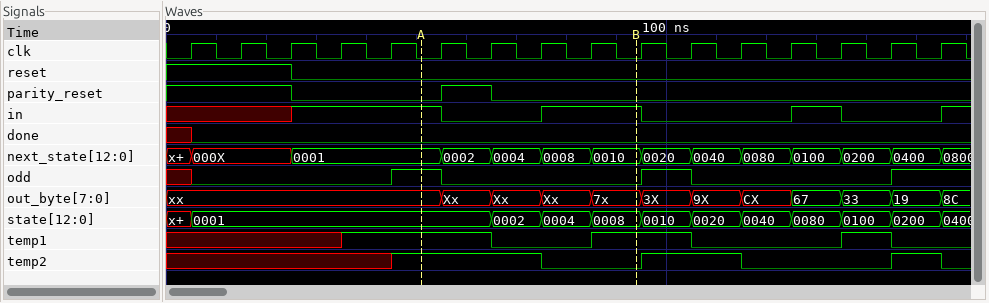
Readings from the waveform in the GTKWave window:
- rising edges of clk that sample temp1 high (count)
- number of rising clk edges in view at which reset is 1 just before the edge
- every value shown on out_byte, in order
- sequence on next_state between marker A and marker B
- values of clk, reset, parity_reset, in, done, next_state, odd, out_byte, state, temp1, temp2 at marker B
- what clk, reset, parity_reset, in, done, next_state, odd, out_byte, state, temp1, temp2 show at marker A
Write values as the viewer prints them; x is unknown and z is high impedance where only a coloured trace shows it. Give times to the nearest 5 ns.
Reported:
6
3
xx, Xx, Xx, Xx, 7x, 3X, 9X, CX, 67, 33, 19, 8C
0001, 0002, 0004, 0008, 0010
clk=0, reset=0, parity_reset=0, in=1, done=0, next_state=0010, odd=0, out_byte=7x, state=0008, temp1=1, temp2=0
clk=0, reset=0, parity_reset=0, in=1, done=0, next_state=0001, odd=1, out_byte=xx, state=0001, temp1=1, temp2=1
